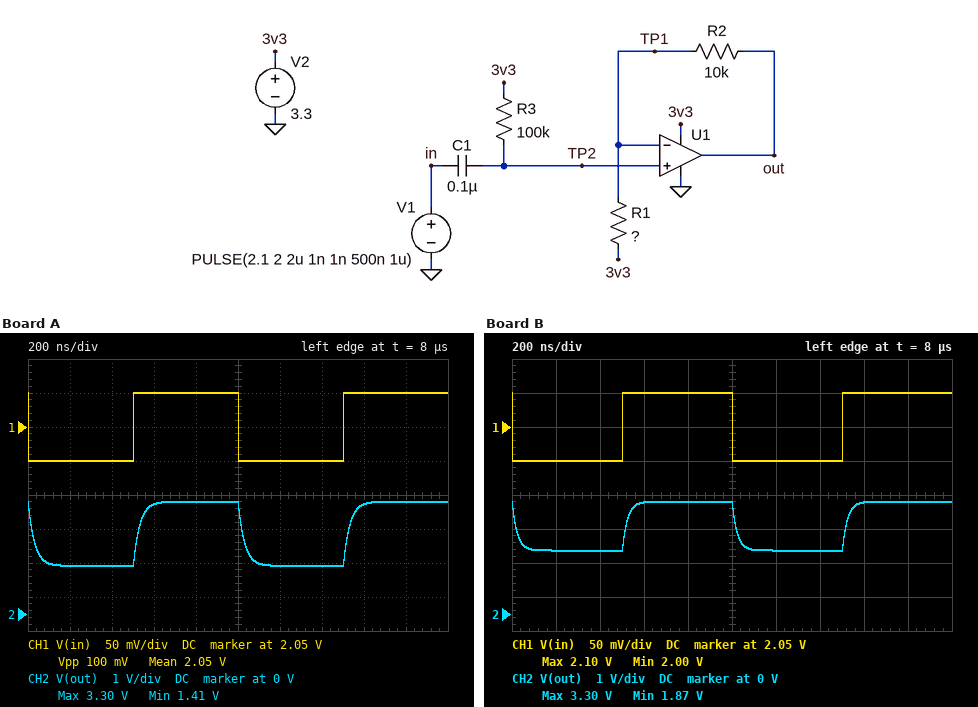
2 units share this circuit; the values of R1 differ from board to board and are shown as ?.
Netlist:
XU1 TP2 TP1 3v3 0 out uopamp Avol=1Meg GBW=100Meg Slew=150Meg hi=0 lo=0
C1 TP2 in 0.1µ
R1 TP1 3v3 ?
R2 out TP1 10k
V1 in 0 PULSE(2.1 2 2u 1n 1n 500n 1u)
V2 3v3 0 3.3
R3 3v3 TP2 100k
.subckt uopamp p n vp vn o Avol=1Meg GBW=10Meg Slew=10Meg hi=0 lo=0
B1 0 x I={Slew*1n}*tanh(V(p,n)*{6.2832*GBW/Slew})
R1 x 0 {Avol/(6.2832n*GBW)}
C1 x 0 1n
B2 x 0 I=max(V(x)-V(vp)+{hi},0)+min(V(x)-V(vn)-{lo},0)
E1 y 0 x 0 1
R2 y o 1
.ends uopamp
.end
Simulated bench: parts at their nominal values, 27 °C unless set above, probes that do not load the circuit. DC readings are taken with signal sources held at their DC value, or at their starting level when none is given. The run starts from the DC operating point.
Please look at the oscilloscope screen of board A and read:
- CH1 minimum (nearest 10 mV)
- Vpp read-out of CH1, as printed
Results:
2.00 V
100 mV
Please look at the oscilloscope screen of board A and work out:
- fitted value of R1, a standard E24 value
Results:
560 Ω
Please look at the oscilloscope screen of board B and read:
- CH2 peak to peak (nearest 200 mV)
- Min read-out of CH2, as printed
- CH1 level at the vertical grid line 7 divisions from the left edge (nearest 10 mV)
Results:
1.4 V
1.87 V
2.00 V
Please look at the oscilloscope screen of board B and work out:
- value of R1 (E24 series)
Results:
750 Ω
